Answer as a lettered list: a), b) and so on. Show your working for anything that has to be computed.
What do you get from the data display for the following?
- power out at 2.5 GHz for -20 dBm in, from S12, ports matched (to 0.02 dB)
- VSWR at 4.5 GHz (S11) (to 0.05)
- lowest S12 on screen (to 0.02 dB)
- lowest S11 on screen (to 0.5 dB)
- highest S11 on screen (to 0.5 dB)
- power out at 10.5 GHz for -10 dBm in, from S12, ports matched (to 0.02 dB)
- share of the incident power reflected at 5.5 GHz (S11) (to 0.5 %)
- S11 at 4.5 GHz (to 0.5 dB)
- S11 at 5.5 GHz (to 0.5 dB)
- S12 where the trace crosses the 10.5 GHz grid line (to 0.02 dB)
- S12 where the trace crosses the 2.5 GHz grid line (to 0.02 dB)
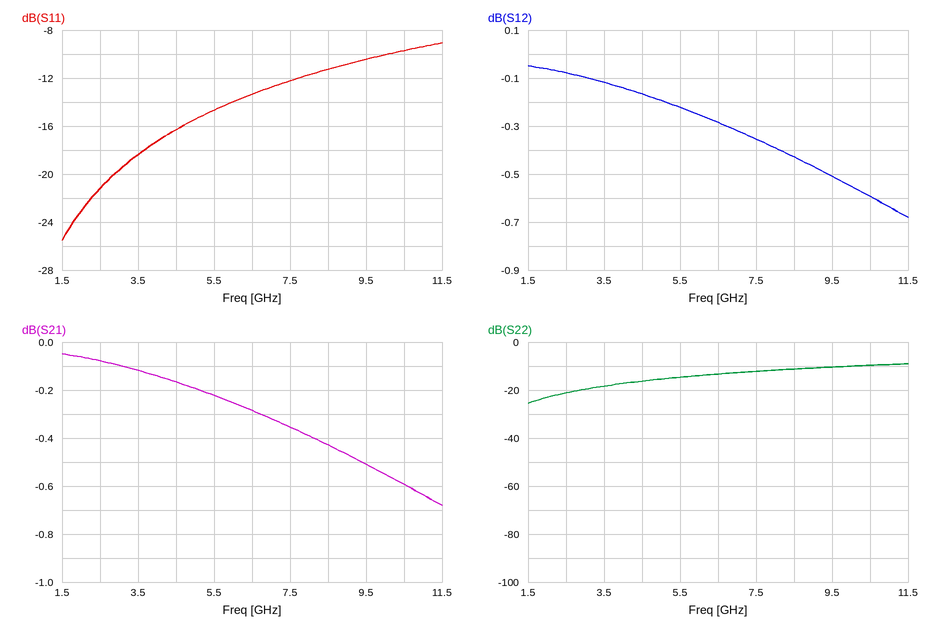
a) -20 dBm + (-0.08 dB) = -20.08 dBm
b) |Γ| = 10^(-16.5/20) = 0.1496; VSWR = (1 + 0.1496)/(1 − 0.1496) ≈ 1.35
c) -0.68 dB
d) -25.5 dB
e) -9.0 dB
f) -10 dBm + (-0.60 dB) = -10.60 dBm
g) 10^(-14.5/10) ≈ 3.5 %
h) -16.5 dB
i) -14.5 dB
j) -0.60 dB
k) -0.08 dB
